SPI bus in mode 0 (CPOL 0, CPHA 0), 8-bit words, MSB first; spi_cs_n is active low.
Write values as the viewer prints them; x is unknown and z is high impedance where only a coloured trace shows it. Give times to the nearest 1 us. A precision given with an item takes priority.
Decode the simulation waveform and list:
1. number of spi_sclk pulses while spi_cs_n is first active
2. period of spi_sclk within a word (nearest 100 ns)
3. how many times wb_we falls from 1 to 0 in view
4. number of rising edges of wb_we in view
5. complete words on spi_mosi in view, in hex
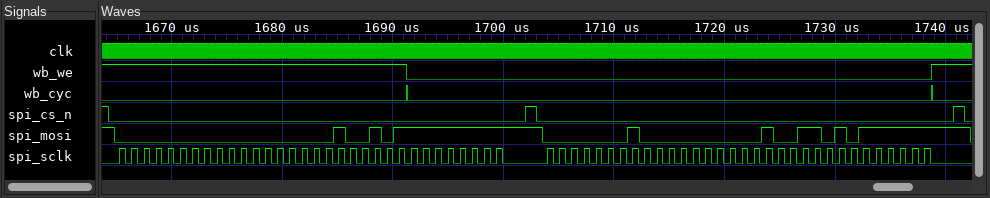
32
1100 ns
1
1
00, 00, 25, FF, 01, 00, 26, BF
